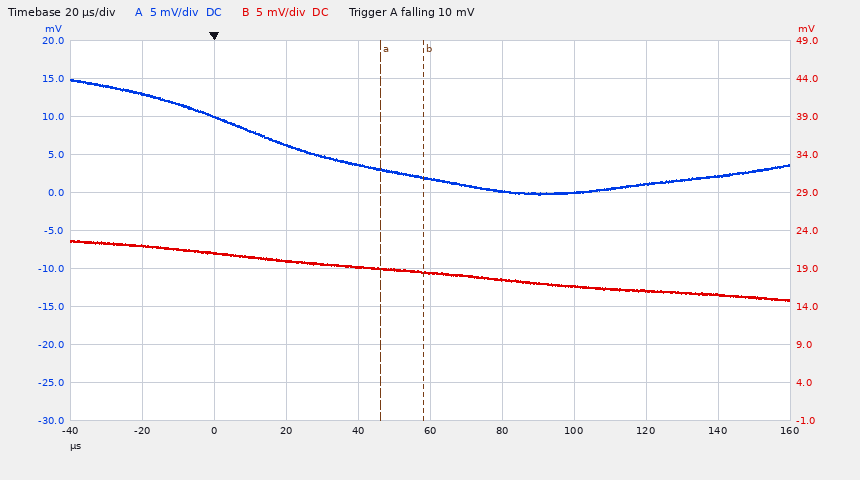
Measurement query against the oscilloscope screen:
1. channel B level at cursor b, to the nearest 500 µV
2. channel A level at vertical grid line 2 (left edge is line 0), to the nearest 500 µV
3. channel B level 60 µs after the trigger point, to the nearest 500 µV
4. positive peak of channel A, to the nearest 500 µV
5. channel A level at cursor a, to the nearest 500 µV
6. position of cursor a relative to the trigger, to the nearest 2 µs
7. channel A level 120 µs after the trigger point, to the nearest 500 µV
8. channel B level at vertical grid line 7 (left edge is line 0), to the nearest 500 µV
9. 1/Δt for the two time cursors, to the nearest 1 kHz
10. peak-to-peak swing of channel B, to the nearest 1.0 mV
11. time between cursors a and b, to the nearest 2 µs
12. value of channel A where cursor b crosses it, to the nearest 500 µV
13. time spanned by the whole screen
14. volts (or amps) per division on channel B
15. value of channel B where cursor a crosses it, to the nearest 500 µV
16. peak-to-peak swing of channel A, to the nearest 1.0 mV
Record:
18.5 mV
10.0 mV
18.5 mV
15.0 mV
3.0 mV
+46 µs
1.0 mV
16.5 mV
83 kHz
8.0 mV
12 µs
2.0 mV
200 µs
5 mV
19.0 mV
15.0 mV
